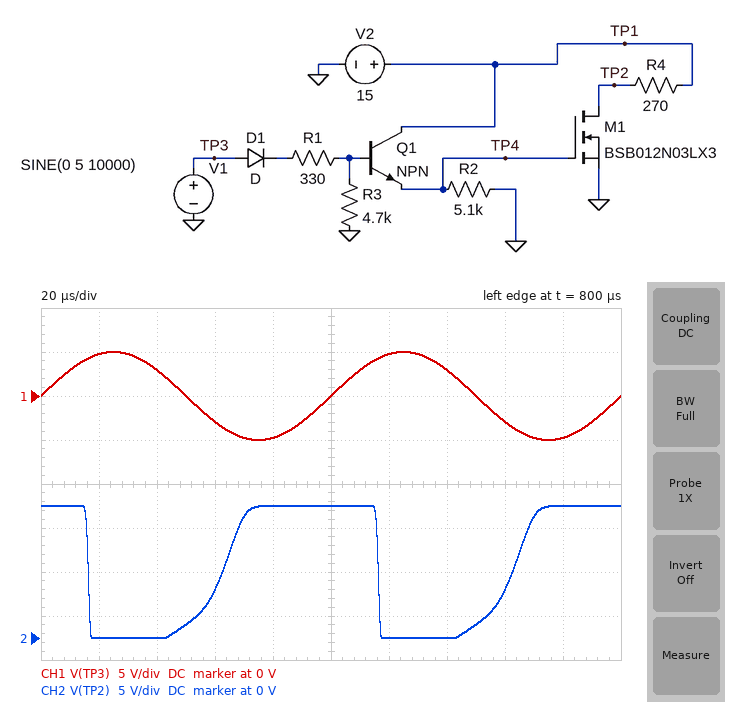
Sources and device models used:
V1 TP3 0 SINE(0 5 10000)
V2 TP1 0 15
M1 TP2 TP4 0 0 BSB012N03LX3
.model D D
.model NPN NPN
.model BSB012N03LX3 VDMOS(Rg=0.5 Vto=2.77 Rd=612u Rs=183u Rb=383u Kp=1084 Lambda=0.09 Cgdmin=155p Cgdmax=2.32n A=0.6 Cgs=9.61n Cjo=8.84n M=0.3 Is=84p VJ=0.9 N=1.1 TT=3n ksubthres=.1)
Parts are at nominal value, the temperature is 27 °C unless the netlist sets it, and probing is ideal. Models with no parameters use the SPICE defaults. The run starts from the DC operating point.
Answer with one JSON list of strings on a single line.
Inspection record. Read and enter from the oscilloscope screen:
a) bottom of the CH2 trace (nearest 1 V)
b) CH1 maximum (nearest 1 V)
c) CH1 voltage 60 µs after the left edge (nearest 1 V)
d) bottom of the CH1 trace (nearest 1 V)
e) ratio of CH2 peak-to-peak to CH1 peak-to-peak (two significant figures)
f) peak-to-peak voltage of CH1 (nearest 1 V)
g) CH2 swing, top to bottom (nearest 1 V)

["0 V", "5 V", "-3 V", "-5 V", "1.5", "10 V", "15 V"]
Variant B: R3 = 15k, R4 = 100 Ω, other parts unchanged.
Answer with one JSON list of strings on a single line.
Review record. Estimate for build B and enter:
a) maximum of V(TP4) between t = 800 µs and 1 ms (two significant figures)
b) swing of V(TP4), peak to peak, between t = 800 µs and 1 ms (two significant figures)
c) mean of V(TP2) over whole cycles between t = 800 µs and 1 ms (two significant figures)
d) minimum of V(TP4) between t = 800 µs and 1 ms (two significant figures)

["3.5 V", "2.3 V", "7.8 V", "1.2 V"]
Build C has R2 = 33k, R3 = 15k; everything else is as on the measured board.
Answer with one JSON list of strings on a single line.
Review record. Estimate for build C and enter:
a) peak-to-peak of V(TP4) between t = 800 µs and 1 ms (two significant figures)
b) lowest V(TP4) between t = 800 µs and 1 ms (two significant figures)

["720 mV", "2.8 V"]
